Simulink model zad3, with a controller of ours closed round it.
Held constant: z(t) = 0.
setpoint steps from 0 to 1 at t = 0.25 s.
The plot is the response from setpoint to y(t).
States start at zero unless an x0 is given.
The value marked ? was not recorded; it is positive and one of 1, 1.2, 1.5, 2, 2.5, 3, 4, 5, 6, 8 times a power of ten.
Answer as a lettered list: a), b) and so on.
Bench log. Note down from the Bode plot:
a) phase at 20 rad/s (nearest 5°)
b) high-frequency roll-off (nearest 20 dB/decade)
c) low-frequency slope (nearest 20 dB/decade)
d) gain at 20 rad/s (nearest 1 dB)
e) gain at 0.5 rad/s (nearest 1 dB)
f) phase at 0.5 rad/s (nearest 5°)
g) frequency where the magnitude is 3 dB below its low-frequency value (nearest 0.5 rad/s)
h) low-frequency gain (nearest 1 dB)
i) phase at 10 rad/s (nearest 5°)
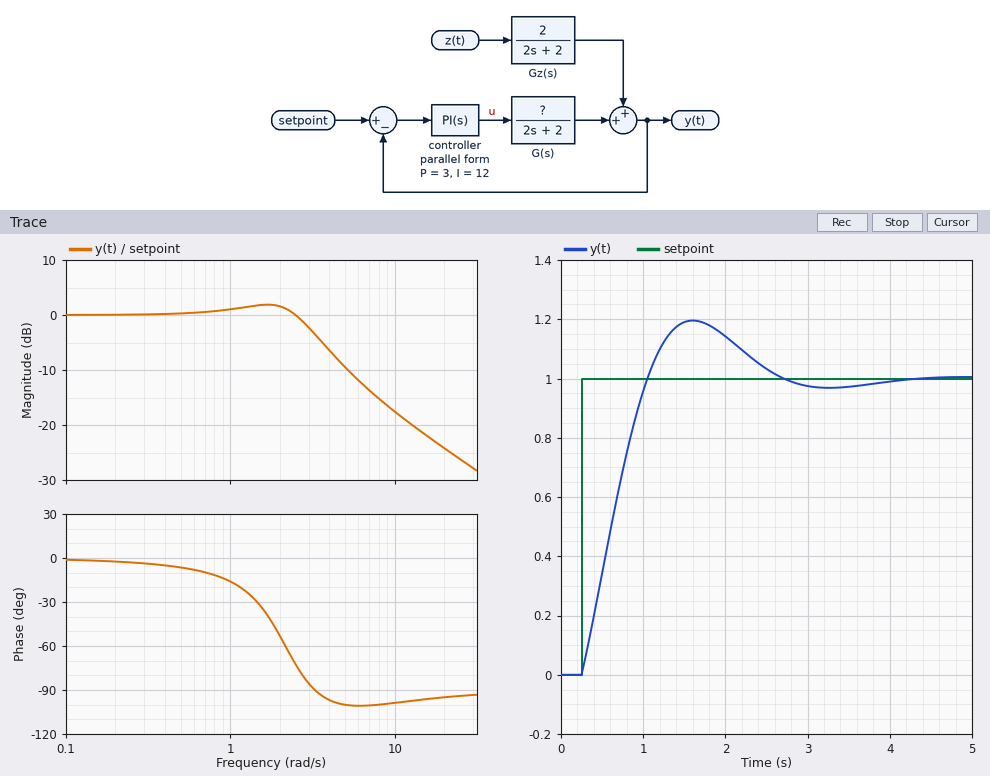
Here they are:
a) -95°
b) -20 dB/decade
c) 0 dB/decade
d) -24 dB
e) 0 dB
f) -5°
g) 3.0 rad/s
h) 0 dB
i) -100°
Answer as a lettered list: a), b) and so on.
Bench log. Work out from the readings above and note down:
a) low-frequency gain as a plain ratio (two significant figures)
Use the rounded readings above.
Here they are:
a) 1.0
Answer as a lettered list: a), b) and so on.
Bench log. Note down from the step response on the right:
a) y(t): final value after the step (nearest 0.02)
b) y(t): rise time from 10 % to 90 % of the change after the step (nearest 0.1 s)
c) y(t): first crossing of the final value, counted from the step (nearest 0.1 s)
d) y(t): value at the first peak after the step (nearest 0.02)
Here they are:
a) 1.00
b) 0.6 s
c) 0.8 s
d) 1.20
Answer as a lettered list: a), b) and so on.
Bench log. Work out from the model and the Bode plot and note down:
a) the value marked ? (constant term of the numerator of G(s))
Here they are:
a) 0.8
